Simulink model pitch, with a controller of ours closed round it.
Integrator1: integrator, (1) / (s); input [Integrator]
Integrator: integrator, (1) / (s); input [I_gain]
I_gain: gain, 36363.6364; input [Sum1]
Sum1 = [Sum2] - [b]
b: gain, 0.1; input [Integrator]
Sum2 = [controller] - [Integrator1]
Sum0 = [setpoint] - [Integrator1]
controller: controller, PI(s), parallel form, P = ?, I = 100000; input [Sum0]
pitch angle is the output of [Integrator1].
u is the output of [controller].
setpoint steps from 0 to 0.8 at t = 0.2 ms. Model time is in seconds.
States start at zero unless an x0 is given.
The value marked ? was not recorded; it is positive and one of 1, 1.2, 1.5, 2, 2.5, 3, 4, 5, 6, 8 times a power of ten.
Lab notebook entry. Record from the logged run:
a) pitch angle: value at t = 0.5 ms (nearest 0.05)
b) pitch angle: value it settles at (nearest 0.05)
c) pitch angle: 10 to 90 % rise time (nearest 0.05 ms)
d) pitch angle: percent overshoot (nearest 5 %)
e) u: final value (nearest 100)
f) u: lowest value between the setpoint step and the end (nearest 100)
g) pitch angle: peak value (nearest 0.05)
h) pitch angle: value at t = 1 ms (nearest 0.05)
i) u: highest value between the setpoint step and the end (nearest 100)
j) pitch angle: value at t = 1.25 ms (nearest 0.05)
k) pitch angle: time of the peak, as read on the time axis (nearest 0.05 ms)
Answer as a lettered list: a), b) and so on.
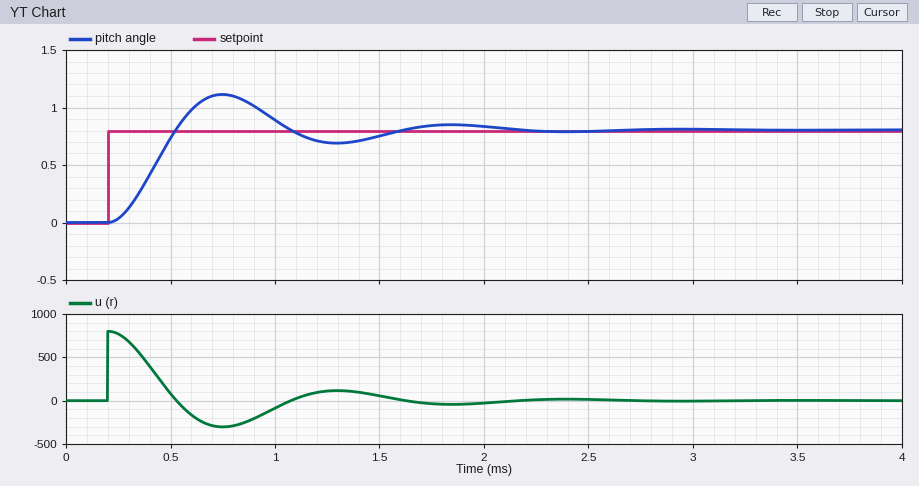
a) 0.75
b) 0.80
c) 0.20 ms
d) 40 %
e) 0
f) -300
g) 1.10
h) 0.90
i) 800
j) 0.70
k) 0.75 ms
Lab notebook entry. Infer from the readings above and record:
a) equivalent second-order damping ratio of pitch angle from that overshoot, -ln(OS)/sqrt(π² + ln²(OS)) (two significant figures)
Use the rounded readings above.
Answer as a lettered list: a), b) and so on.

a) 0.28
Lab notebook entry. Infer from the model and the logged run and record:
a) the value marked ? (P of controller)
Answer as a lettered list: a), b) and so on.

a) 1000
